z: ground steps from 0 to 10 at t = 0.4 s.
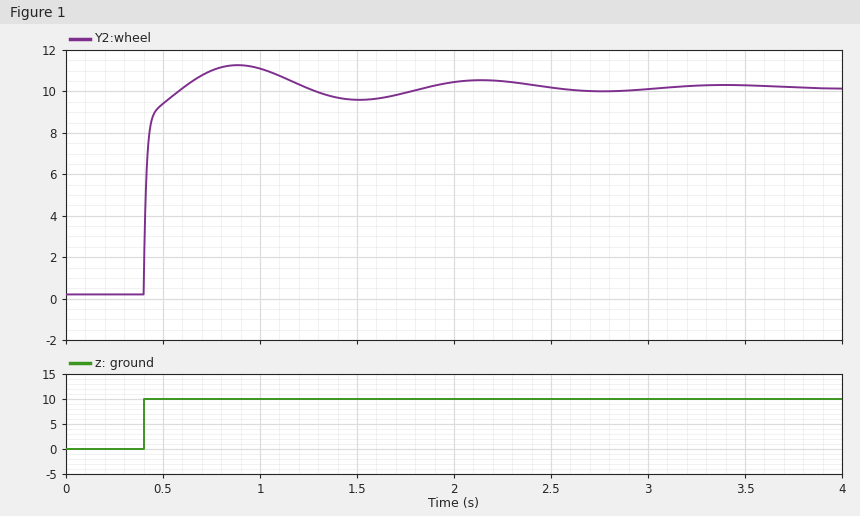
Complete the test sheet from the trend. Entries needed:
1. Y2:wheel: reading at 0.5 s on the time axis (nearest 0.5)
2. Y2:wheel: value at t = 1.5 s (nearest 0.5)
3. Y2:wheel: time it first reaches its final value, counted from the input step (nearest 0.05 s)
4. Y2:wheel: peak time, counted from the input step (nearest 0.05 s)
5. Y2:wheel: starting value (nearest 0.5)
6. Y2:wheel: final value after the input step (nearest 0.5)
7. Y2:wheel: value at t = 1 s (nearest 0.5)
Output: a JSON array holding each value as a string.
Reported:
["9.5", "9.5", "0.20 s", "0.50 s", "0.0", "10.0", "11.0"]
